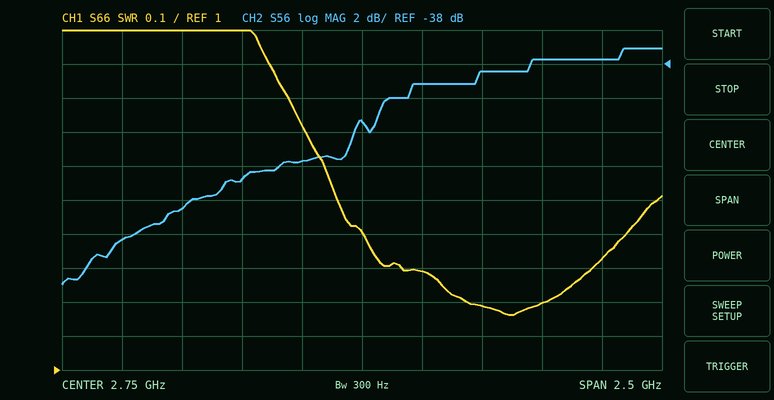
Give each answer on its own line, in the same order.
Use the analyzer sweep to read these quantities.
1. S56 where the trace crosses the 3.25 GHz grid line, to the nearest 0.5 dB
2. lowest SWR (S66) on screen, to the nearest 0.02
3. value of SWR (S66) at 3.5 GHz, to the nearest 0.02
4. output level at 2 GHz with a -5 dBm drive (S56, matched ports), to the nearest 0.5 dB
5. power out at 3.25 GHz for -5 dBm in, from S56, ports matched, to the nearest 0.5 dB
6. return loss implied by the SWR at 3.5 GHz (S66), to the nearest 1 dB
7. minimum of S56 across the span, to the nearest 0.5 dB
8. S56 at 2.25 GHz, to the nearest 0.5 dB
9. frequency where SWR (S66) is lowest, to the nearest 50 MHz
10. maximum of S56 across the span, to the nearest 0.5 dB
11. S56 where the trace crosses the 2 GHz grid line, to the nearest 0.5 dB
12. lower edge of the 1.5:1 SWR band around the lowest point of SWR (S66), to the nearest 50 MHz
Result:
-38.5 dB
1.16
1.20
-51.5 dBm
-43.5 dBm
21 dB
-51.0 dB
-45.0 dB
3.35 GHz
-37.0 dB
-46.5 dB
2.65 GHz
